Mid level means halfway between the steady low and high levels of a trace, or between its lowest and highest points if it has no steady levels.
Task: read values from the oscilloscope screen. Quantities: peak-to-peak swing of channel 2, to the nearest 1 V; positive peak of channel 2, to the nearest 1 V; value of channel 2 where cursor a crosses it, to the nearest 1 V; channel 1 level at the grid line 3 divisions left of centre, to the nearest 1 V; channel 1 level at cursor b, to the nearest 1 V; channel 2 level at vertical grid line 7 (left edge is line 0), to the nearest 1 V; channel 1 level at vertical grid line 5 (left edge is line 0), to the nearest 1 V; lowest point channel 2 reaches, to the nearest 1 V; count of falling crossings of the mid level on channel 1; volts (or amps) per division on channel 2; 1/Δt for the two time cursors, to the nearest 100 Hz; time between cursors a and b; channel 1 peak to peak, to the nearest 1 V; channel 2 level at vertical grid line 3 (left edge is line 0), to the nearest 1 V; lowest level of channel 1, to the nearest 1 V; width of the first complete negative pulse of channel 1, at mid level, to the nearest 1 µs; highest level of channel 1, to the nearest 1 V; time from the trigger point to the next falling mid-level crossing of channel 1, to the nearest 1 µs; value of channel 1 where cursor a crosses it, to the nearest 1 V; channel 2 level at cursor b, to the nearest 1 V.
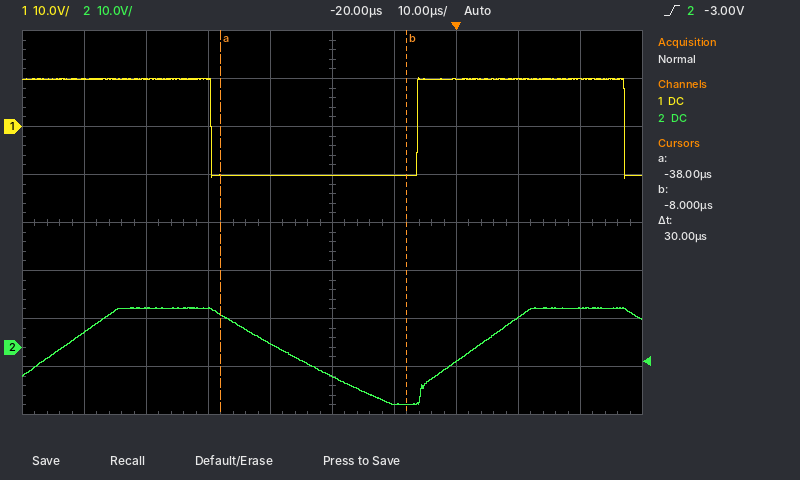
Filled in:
20 V
8 V
7 V
10 V
-10 V
-3 V
-10 V
-12 V
2
10 V
33.3 kHz
30 µs
21 V
8 V
-11 V
33 µs
10 V
27 µs
-10 V
-12 V
